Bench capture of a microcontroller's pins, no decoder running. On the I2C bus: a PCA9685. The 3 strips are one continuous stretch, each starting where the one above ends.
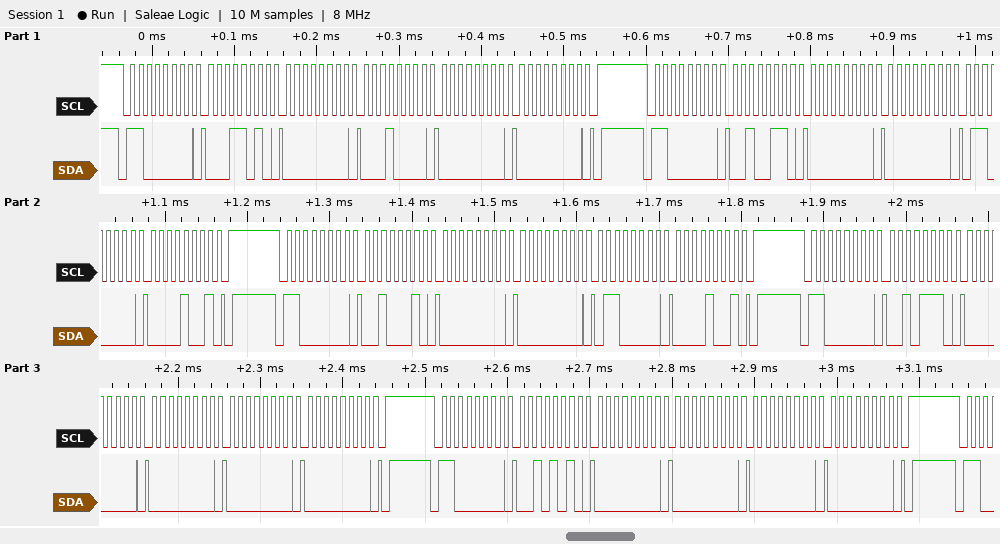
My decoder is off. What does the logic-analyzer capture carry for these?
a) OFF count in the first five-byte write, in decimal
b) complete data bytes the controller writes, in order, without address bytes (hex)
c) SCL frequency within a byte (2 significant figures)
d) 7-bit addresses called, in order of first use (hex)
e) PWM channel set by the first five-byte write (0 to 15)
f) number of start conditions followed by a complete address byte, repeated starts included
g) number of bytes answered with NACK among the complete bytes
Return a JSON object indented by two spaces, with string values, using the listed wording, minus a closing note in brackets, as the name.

{
  "OFF count in the first five-byte write, in decimal": "0",
  "complete data bytes the controller writes, in order, without address bytes": "1A 00 10 00 00 26 00 00 60 09 22 00 00 60 09 2E 00 00 00 00 2A 00 00 00 00",
  "SCL frequency within a byte": "100 kHz",
  "7-bit addresses called, in order of first use": "0x60",
  "PWM channel set by the first five-byte write": "5",
  "number of start conditions followed by a complete address byte, repeated starts included": "5",
  "number of bytes answered with NACK among the complete bytes": "0"
}
